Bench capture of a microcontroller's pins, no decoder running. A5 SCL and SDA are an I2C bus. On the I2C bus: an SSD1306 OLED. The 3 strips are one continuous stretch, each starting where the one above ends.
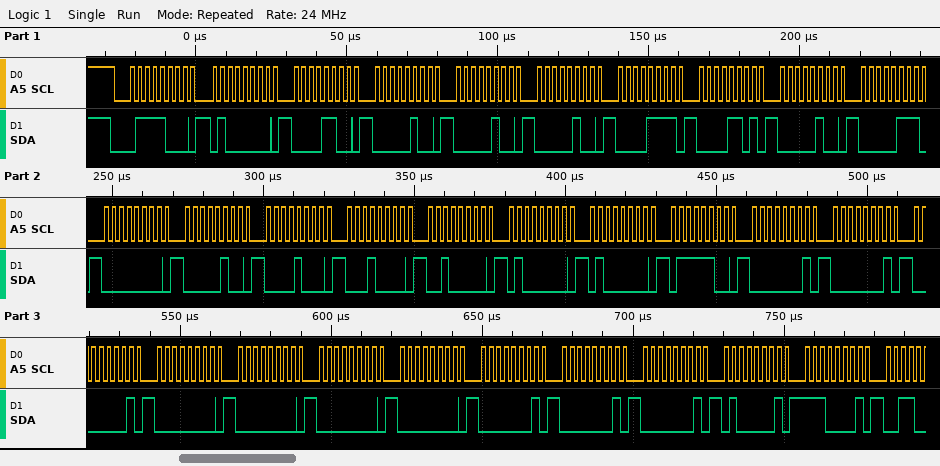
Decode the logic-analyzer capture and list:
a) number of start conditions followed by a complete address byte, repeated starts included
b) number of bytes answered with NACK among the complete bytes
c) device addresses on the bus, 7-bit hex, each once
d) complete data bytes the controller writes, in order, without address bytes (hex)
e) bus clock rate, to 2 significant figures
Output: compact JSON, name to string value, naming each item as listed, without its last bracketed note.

{"number of start conditions followed by a complete address byte, repeated starts included": "1", "number of bytes answered with NACK among the complete bytes": "0", "device addresses on the bus, 7-bit hex, each once": "0x3C", "complete data bytes the controller writes, in order, without address bytes": "40 0C 04 04 04 0F 0D 04 07 00 04 08 10 20 40 40 7C 01 01 01 00 00 00 00 01 01 01 41 E1", "bus clock rate, to 2 significant figures": "400 kHz"}
